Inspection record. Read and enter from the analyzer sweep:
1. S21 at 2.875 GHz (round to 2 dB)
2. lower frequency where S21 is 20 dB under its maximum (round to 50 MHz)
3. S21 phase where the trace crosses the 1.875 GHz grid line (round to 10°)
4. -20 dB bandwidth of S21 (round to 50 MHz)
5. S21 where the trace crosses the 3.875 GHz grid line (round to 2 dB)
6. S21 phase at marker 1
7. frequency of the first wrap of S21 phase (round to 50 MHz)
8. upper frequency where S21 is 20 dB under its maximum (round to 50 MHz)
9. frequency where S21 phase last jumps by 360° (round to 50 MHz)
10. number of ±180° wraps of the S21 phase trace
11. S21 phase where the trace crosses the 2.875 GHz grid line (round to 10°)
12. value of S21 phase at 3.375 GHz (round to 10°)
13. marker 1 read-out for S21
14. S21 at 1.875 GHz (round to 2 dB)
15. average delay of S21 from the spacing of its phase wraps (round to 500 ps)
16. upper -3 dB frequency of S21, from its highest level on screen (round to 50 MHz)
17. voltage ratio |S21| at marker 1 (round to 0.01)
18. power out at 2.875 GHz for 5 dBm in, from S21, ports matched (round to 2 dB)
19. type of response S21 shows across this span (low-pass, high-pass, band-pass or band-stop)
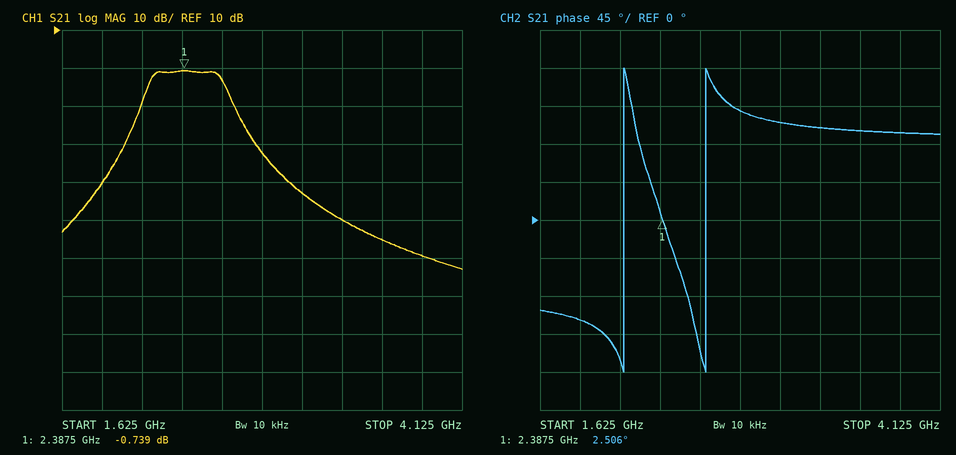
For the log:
-22 dB
2.00 GHz
-120°
850 MHz
-50 dB
2.506°
2.15 GHz
2.85 GHz
2.65 GHz
2
130°
110°
-0.739 dB
-30 dB
2.0 ns
2.65 GHz
0.92
-18 dBm
band-pass
